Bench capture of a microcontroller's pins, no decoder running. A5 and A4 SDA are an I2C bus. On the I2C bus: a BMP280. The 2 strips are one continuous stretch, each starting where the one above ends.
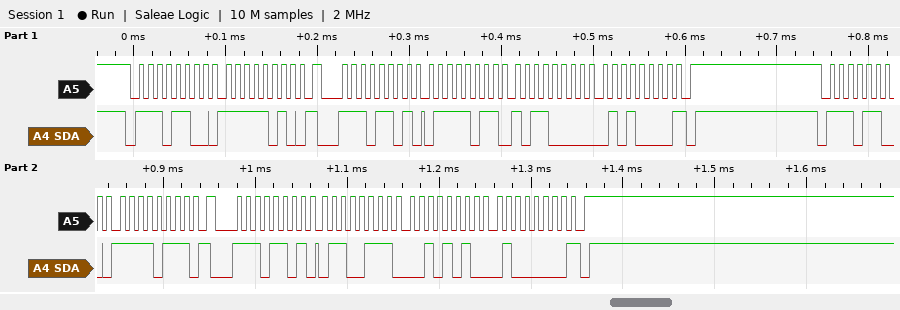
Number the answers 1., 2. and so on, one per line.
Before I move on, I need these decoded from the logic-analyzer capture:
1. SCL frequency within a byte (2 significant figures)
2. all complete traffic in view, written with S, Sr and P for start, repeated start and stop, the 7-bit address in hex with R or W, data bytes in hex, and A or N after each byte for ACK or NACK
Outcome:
1. 100 kHz
2. S 76W A FA A Sr 76R A 7B A B0 A 50 N P S 76W A F7 A Sr 76R A 67 A 2A A 40 N P
